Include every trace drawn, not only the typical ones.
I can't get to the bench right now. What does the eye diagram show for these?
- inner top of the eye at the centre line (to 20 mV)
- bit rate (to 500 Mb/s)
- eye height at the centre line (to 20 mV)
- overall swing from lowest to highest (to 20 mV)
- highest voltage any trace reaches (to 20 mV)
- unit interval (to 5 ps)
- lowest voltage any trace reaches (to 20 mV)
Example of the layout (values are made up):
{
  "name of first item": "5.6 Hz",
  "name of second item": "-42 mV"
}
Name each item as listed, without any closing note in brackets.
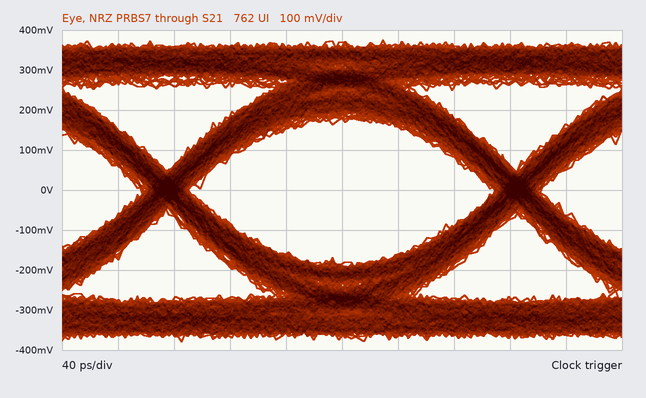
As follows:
{
  "inner top of the eye at the centre line": "180 mV",
  "bit rate": "4.0 Gb/s",
  "eye height at the centre line": "360 mV",
  "overall swing from lowest to highest": "760 mV",
  "highest voltage any trace reaches": "380 mV",
  "unit interval": "250 ps",
  "lowest voltage any trace reaches": "-380 mV"
}
